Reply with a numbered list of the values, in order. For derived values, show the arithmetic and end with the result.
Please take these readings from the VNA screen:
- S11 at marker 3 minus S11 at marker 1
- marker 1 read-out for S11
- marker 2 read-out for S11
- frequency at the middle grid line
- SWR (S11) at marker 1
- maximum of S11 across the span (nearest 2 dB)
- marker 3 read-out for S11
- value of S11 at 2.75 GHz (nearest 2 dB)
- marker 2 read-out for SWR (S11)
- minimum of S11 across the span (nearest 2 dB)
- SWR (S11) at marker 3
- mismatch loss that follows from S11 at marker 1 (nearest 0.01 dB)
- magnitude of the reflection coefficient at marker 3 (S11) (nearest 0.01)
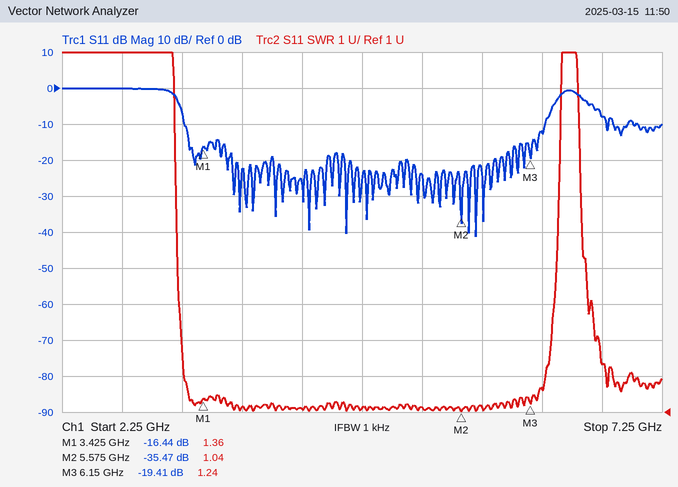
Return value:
1. -19.41 − (-16.44) = -2.97 dB
2. -16.44 dB
3. -35.47 dB
4. 4.75 GHz
5. 1.36
6. 0 dB
7. -19.41 dB
8. 0 dB
9. 1.04
10. -42 dB
11. 1.24
12. −10 log10(1 − 10^(-16.44/10)) ≈ 0.10 dB
13. 10^(-19.41/20) ≈ 0.11
